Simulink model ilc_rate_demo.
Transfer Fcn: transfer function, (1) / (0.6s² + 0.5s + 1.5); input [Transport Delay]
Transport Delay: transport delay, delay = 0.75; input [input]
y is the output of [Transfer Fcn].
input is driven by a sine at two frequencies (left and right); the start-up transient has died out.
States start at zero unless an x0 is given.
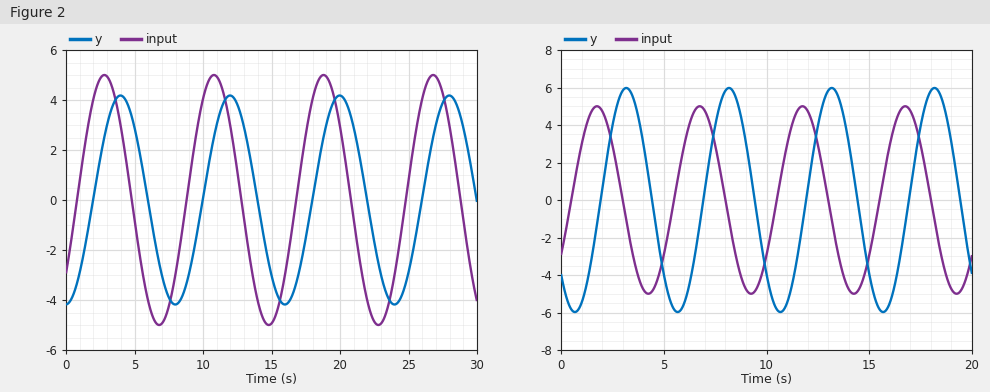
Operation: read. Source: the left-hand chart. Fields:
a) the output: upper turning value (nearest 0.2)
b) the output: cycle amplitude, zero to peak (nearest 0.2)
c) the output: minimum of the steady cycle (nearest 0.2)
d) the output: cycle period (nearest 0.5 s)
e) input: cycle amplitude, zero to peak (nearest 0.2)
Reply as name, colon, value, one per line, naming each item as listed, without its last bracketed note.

the output: upper turning value: 4.2
the output: cycle amplitude, zero to peak: 4.2
the output: minimum of the steady cycle: -4.2
the output: cycle period: 8.0 s
input: cycle amplitude, zero to peak: 5.0
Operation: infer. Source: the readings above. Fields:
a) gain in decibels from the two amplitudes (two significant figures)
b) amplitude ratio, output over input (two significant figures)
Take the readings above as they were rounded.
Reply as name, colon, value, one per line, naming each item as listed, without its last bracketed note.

gain in decibels from the two amplitudes: -1.5 dB
amplitude ratio, output over input: 0.84
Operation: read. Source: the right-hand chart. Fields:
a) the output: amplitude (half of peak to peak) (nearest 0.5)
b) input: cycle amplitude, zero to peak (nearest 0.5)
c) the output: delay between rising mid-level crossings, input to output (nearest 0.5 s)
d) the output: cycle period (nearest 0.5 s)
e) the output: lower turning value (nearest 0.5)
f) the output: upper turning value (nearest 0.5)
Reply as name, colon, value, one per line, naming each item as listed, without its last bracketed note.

the output: amplitude (half of peak to peak): 6.0
input: cycle amplitude, zero to peak: 5.0
the output: delay between rising mid-level crossings, input to output: 1.5 s
the output: cycle period: 5.0 s
the output: lower turning value: -6.0
the output: upper turning value: 6.0
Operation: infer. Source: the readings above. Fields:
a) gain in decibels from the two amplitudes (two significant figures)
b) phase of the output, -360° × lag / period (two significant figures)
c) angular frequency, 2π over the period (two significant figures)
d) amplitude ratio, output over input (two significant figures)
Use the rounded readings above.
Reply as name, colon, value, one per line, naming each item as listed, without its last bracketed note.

gain in decibels from the two amplitudes: 1.6 dB
phase of the output, -360° × lag / period: -110°
angular frequency, 2π over the period: 1.3 rad/s
amplitude ratio, output over input: 1.2
